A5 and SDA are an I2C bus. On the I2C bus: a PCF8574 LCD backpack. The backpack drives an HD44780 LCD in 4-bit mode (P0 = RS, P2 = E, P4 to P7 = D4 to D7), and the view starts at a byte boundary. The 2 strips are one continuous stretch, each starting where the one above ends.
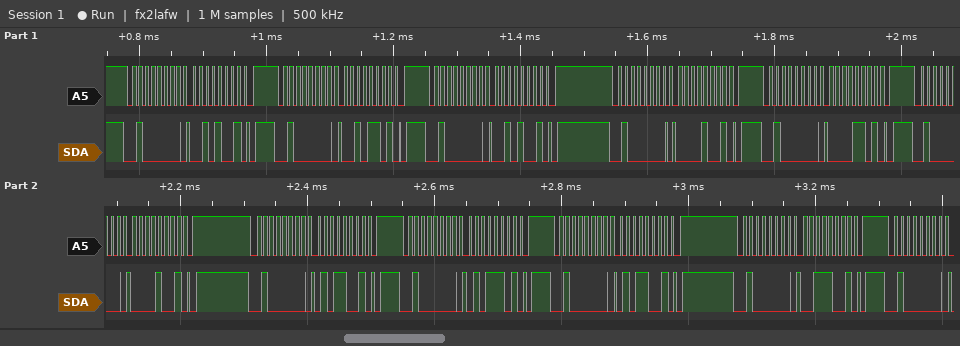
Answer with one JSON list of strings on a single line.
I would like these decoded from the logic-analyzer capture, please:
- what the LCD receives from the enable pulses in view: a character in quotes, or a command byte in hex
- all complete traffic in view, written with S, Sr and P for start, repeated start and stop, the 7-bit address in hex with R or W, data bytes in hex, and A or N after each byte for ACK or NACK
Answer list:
["' '", "S 20W A 29 A P S 20W A 2D A P S 20W A 29 A P S 20W A 09 A P S 20W A 0D A P S 20W A 09 A P S 20W A 59 A P S 20W A 5D A P S 20W A 59 A P S 20W A 39 A P S 20W A"]
